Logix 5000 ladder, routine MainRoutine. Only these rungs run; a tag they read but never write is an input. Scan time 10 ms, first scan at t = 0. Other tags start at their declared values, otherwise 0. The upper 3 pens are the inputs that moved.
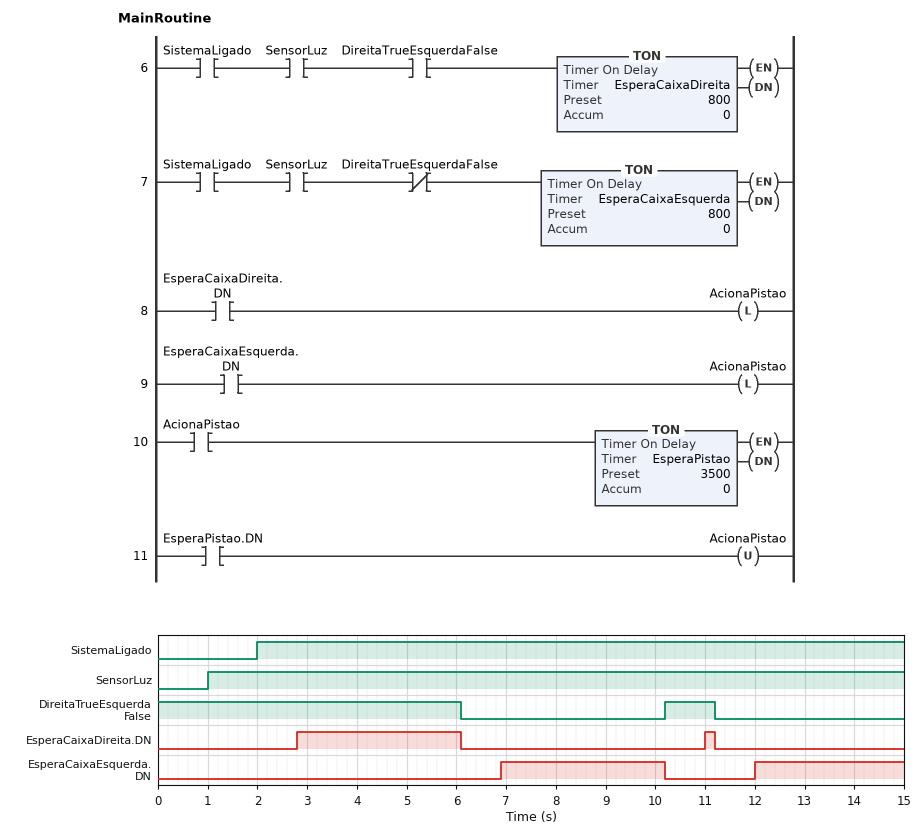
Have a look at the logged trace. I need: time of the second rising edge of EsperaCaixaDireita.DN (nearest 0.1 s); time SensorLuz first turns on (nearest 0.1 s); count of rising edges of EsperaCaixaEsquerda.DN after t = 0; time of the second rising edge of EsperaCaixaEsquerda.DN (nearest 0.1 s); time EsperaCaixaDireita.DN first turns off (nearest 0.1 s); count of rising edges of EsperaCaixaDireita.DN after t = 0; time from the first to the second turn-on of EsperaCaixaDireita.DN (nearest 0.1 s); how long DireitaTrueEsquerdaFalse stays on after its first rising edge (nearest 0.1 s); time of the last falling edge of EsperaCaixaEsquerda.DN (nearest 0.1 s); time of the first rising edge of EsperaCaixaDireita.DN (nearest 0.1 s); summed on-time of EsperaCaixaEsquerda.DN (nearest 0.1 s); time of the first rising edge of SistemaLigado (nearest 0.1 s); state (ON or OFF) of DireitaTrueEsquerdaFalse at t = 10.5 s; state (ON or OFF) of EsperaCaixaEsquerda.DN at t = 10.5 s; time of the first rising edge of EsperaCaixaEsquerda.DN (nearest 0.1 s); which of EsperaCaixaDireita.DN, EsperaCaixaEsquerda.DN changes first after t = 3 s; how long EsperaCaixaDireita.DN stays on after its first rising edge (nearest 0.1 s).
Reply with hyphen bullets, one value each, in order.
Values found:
- 11.0 s
- 1.0 s
- 2
- 12.0 s
- 6.1 s
- 2
- 8.2 s
- 1.0 s
- 10.2 s
- 2.8 s
- 6.3 s
- 2.0 s
- ON
- OFF
- 6.9 s
- EsperaCaixaDireita.DN
- 3.3 s
